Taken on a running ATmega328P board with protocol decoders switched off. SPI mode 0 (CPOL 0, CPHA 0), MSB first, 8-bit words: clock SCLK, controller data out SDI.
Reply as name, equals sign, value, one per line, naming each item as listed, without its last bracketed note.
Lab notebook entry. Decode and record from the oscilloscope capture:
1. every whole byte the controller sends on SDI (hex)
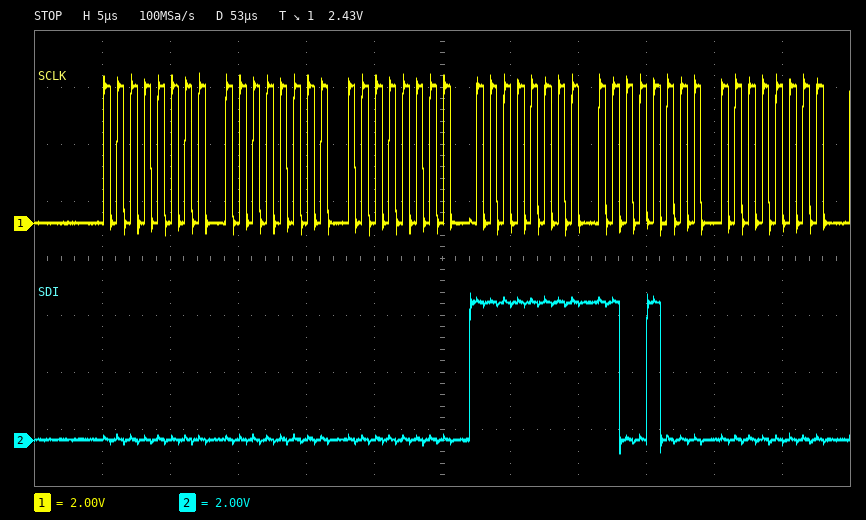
every whole byte the controller sends on SDI = 0x00 0x00 0x00 0xFF 0xC8 0x00
